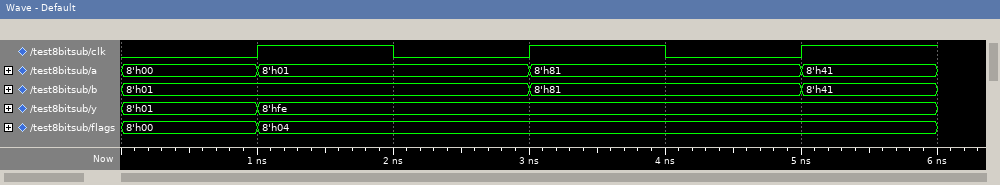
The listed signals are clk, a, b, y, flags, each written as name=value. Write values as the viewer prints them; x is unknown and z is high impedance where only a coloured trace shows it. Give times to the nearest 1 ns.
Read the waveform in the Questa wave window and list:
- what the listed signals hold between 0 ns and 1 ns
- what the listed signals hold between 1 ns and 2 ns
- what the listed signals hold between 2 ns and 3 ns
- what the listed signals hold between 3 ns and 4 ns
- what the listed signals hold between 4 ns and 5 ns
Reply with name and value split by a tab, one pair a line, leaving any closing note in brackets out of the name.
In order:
what the listed signals hold between 0 ns and 1 ns	clk=0, a=8'h00, b=8'h01, y=8'h01, flags=8'h00
what the listed signals hold between 1 ns and 2 ns	clk=1, a=8'h01, b=8'h01, y=8'hfe, flags=8'h04
what the listed signals hold between 2 ns and 3 ns	clk=0, a=8'h01, b=8'h01, y=8'hfe, flags=8'h04
what the listed signals hold between 3 ns and 4 ns	clk=1, a=8'h81, b=8'h81, y=8'hfe, flags=8'h04
what the listed signals hold between 4 ns and 5 ns	clk=0, a=8'h81, b=8'h81, y=8'hfe, flags=8'h04
